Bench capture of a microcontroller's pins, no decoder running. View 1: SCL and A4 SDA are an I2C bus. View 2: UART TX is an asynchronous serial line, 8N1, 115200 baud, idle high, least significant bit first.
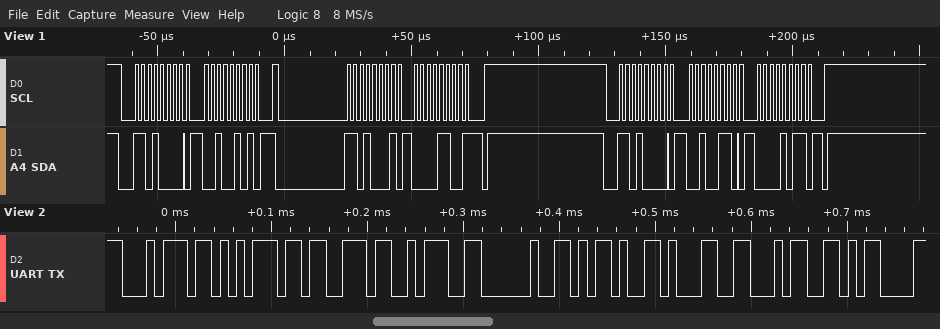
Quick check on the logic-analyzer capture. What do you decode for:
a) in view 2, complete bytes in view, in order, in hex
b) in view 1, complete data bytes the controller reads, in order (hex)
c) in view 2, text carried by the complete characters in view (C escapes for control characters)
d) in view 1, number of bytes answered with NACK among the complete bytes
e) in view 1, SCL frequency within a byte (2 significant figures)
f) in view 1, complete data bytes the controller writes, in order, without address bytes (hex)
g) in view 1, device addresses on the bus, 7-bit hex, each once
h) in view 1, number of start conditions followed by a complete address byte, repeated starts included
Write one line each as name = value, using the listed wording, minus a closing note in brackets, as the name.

in view 2, complete bytes in view, in order, in hex = 0x74 0x75 0x73 0x3A 0x20 0x2D 0x31 0x34 0x0D
in view 1, complete data bytes the controller reads, in order = 0C
in view 2, text carried by the complete characters in view = "tus: -14\r"
in view 1, number of bytes answered with NACK among the complete bytes = 1
in view 1, SCL frequency within a byte = 400 kHz
in view 1, complete data bytes the controller writes, in order, without address bytes = 25 26 0B
in view 1, device addresses on the bus, 7-bit hex, each once = 0x68
in view 1, number of start conditions followed by a complete address byte, repeated starts included = 3
